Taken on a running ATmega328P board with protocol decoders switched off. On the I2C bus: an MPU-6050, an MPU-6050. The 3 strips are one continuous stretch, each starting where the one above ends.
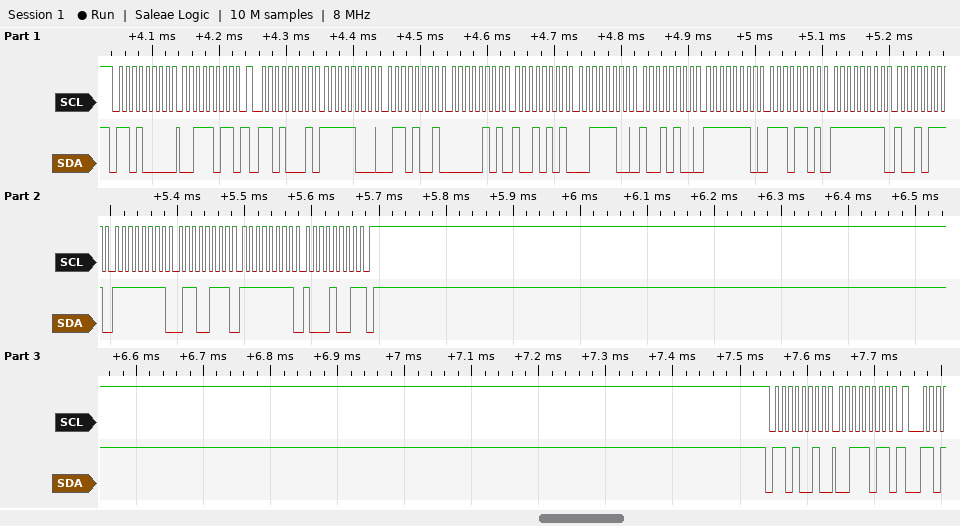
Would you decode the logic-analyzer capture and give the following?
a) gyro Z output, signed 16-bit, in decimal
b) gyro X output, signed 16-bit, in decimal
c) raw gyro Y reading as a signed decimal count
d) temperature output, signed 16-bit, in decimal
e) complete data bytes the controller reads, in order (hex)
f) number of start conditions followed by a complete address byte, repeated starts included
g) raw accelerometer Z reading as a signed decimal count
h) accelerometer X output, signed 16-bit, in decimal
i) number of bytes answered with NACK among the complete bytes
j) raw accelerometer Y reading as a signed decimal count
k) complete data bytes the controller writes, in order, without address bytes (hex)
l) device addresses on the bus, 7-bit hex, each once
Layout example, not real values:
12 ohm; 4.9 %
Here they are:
-119; -105; -153; -275; F8 69 05 95 3C 94 FE ED FF 97 FF 67 FF 89; 3; 15508; -1943; 1; 1429; 3B 3B; 0x68 0x69
